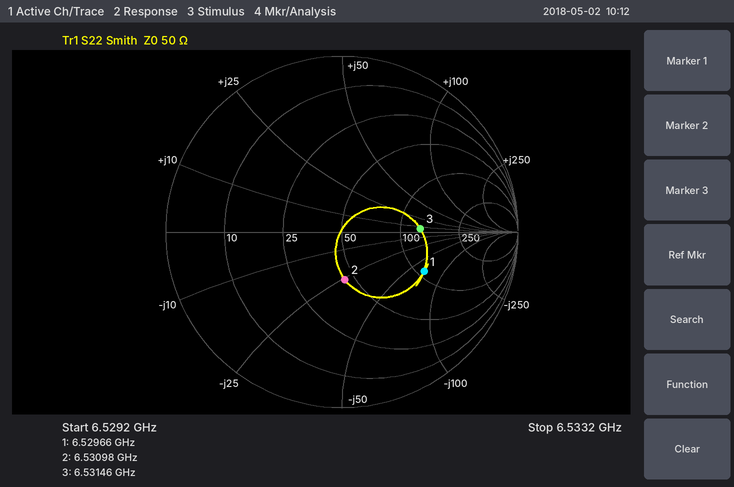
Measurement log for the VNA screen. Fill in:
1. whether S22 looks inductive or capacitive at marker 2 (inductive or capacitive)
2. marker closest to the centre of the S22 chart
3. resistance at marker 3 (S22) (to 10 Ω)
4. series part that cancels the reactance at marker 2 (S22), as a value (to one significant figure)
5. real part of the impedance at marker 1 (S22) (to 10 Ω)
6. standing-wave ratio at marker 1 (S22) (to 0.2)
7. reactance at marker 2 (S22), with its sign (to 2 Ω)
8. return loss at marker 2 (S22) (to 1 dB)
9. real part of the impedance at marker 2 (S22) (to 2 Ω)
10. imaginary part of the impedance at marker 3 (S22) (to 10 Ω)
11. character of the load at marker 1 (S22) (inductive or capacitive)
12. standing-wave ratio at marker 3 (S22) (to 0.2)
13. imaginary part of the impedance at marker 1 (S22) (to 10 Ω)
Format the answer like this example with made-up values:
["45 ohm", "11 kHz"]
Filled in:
["capacitive", "marker 2", "130 Ω", "600 pH", "110 Ω", "3.2", "-26 Ω", "11 dB", "44 Ω", "+10 Ω", "capacitive", "2.6", "-70 Ω"]
